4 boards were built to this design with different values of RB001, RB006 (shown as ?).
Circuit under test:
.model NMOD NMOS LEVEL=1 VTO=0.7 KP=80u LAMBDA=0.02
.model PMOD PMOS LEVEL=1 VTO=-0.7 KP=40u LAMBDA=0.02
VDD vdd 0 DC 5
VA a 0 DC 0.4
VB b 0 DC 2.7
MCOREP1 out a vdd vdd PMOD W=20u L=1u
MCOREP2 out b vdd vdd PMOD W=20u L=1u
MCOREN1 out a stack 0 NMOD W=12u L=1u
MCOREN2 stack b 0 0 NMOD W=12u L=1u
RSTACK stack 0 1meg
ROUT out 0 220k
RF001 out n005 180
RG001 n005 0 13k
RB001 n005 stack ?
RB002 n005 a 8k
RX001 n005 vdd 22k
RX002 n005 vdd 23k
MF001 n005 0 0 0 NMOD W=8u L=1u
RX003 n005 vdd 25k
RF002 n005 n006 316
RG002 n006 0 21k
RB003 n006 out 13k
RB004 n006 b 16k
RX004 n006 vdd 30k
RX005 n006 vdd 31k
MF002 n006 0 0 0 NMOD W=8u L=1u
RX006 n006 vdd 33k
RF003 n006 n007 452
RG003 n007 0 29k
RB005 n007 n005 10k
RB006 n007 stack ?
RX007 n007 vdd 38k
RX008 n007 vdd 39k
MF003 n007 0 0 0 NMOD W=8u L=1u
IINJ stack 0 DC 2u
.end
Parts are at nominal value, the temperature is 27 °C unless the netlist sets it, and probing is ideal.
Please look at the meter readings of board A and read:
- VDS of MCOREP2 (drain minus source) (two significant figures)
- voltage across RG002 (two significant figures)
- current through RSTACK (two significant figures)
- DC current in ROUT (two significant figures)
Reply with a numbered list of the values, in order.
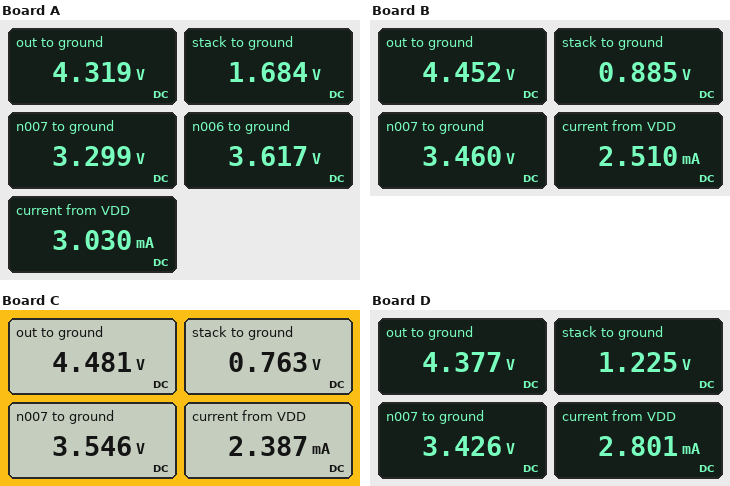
1. -680 mV
2. 3.6 V
3. 1.7 µA
4. 20 µA
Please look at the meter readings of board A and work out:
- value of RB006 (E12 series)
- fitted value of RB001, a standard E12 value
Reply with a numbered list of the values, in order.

1. 2.2 kΩ
2. 1.8 kΩ
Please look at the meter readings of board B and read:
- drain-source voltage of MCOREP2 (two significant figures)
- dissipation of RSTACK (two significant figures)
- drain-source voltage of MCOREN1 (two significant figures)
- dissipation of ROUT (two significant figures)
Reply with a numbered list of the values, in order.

1. -550 mV
2. 780 nW
3. 3.6 V
4. 90 µW
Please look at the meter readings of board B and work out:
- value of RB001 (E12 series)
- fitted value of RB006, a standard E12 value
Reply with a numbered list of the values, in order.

1. 5.6 kΩ
2. 3.3 kΩ
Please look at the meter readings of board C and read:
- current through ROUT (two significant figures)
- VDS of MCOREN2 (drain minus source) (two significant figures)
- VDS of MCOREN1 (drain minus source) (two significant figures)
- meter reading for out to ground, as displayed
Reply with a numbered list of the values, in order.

1. 20 µA
2. 760 mV
3. 3.7 V
4. 4.481 V
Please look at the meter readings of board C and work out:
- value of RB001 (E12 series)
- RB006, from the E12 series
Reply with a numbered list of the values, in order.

1. 6.8 kΩ
2. 3.9 kΩ
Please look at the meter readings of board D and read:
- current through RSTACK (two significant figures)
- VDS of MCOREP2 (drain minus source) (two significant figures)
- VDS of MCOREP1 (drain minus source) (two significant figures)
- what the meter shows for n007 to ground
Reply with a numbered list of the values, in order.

1. 1.2 µA
2. -620 mV
3. -620 mV
4. 3.426 V
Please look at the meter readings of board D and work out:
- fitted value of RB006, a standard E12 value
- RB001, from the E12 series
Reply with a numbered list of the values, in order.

1. 3.3 kΩ
2. 2.7 kΩ
